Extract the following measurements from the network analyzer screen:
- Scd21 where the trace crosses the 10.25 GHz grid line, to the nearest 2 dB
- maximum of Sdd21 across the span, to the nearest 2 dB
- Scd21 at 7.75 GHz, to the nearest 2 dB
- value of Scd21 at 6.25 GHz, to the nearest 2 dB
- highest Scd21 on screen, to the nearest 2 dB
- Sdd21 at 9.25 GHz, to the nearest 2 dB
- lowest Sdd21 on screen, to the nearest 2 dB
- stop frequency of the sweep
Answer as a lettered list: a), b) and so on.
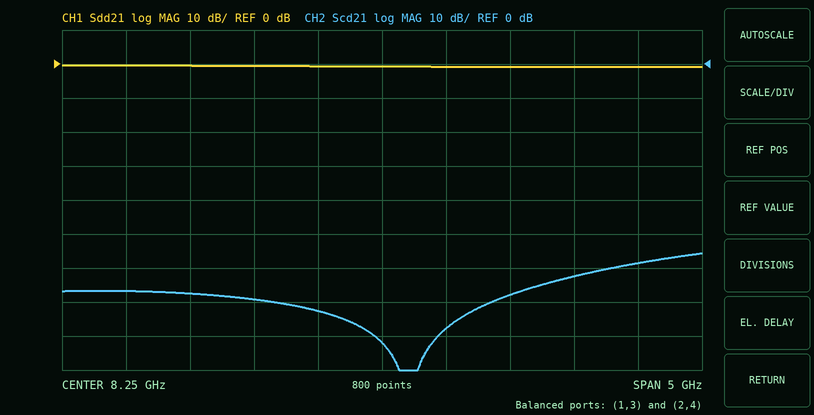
a) -58 dB
b) 0 dB
c) -72 dB
d) -66 dB
e) -56 dB
f) 0 dB
g) 0 dB
h) 10.75 GHz
